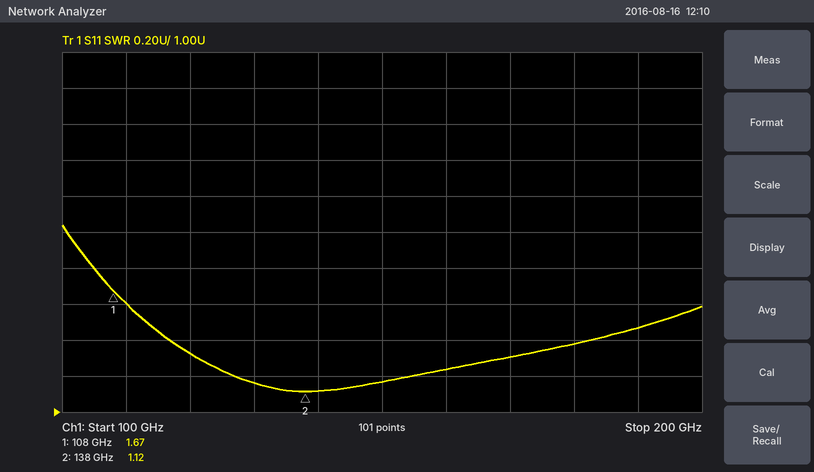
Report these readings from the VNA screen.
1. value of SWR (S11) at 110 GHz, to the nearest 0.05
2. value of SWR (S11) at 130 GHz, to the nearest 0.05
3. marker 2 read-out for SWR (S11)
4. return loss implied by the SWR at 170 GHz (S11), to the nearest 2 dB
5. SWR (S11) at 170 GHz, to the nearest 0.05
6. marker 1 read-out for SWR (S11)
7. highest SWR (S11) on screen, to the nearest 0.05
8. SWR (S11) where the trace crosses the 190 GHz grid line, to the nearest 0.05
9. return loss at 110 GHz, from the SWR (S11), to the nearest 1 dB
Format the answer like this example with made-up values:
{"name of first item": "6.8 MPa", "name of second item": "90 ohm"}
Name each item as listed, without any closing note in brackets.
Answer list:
{"value of SWR (S11) at 110 GHz, to the nearest 0.05": "1.60", "value of SWR (S11) at 130 GHz, to the nearest 0.05": "1.15", "marker 2 read-out for SWR": "1.12", "return loss implied by the SWR at 170 GHz (S11), to the nearest 2 dB": "18 dB", "SWR (S11) at 170 GHz, to the nearest 0.05": "1.30", "marker 1 read-out for SWR": "1.67", "highest SWR (S11) on screen, to the nearest 0.05": "2.05", "SWR (S11) where the trace crosses the 190 GHz grid line, to the nearest 0.05": "1.45", "return loss at 110 GHz, from the SWR (S11), to the nearest 1 dB": "13 dB"}
